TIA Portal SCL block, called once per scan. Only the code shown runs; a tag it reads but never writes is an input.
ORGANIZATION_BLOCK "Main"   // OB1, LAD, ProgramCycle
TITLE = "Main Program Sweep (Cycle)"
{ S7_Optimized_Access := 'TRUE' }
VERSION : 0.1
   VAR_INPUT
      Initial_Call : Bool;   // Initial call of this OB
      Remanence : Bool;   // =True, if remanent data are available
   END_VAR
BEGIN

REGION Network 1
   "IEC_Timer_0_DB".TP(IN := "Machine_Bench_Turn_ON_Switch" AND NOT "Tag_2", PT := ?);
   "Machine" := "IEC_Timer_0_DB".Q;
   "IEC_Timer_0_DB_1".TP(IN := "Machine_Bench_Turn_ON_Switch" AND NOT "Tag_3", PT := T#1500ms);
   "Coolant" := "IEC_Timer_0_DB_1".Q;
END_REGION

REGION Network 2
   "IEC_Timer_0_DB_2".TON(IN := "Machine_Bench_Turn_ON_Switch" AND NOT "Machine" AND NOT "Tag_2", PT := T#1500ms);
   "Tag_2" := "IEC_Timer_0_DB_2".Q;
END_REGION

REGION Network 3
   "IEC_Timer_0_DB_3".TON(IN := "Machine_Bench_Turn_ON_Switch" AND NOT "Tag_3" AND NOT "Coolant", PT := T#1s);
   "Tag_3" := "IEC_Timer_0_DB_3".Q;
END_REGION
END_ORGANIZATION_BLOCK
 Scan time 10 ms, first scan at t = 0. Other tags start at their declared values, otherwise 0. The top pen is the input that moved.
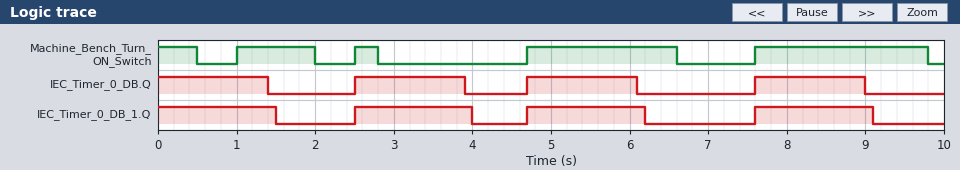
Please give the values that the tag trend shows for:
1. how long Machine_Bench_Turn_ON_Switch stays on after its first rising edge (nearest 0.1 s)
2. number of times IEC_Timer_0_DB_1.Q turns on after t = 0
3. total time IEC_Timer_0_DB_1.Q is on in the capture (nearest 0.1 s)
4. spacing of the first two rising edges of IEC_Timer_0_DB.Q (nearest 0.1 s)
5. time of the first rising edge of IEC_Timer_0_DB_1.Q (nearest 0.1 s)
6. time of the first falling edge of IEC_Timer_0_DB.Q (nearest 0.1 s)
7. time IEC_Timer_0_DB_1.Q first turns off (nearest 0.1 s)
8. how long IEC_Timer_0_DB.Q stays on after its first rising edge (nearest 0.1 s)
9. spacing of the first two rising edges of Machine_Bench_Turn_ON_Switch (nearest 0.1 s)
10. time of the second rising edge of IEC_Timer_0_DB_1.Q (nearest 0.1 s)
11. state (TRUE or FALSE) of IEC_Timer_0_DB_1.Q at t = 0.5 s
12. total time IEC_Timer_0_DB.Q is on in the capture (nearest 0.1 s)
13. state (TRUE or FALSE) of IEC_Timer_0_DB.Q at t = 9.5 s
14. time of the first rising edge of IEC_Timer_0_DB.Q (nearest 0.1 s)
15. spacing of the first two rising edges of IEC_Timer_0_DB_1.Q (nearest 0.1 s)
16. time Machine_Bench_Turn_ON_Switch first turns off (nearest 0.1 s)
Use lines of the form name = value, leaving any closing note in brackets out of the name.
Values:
how long Machine_Bench_Turn_ON_Switch stays on after its first rising edge = 1.0 s
number of times IEC_Timer_0_DB_1.Q turns on after t = 0 = 3
total time IEC_Timer_0_DB_1.Q is on in the capture = 6.0 s
spacing of the first two rising edges of IEC_Timer_0_DB.Q = 2.2 s
time of the first rising edge of IEC_Timer_0_DB_1.Q = 2.5 s
time of the first falling edge of IEC_Timer_0_DB.Q = 1.4 s
time IEC_Timer_0_DB_1.Q first turns off = 1.5 s
how long IEC_Timer_0_DB.Q stays on after its first rising edge = 1.4 s
spacing of the first two rising edges of Machine_Bench_Turn_ON_Switch = 1.5 s
time of the second rising edge of IEC_Timer_0_DB_1.Q = 4.7 s
state (TRUE or FALSE) of IEC_Timer_0_DB_1.Q at t = 0.5 s = TRUE
total time IEC_Timer_0_DB.Q is on in the capture = 5.6 s
state (TRUE or FALSE) of IEC_Timer_0_DB.Q at t = 9.5 s = FALSE
time of the first rising edge of IEC_Timer_0_DB.Q = 2.5 s
spacing of the first two rising edges of IEC_Timer_0_DB_1.Q = 2.2 s
time Machine_Bench_Turn_ON_Switch first turns off = 0.5 s
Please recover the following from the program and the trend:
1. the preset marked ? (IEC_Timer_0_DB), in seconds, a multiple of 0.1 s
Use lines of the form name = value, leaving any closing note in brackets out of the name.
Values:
the preset marked ? (IEC_Timer_0_DB), in seconds, a multiple of 0.1 s = 1.4 s
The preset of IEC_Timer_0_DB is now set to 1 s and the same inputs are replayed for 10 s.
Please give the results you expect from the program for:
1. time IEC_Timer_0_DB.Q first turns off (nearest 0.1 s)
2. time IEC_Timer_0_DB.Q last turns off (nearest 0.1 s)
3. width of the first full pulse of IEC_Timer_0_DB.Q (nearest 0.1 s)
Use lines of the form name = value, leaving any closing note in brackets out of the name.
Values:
time IEC_Timer_0_DB.Q first turns off = 1.0 s
time IEC_Timer_0_DB.Q last turns off = 8.6 s
width of the first full pulse of IEC_Timer_0_DB.Q = 1.0 s
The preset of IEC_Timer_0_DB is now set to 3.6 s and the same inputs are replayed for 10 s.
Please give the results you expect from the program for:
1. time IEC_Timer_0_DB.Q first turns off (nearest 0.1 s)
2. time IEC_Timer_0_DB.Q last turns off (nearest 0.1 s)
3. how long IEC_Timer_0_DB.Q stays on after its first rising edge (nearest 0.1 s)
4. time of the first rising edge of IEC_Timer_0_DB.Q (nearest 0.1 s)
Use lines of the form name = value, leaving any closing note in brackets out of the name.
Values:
time IEC_Timer_0_DB.Q first turns off = 3.6 s
time IEC_Timer_0_DB.Q last turns off = 8.3 s
how long IEC_Timer_0_DB.Q stays on after its first rising edge = 3.6 s
time of the first rising edge of IEC_Timer_0_DB.Q = 4.7 s
